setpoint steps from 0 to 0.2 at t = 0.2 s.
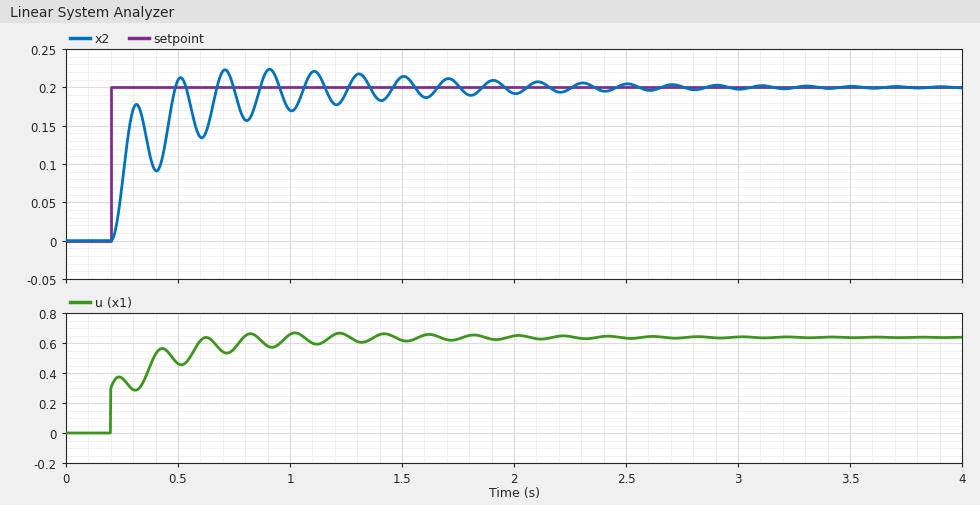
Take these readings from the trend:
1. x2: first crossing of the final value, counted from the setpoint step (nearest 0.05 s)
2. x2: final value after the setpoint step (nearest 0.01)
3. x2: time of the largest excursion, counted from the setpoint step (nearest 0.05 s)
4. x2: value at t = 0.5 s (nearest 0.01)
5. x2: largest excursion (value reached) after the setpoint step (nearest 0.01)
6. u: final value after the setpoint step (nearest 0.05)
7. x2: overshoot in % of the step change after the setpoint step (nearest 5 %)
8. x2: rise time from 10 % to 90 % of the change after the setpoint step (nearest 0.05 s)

0.30 s
0.20
0.70 s
0.21
0.22
0.65
10 %
0.25 s
